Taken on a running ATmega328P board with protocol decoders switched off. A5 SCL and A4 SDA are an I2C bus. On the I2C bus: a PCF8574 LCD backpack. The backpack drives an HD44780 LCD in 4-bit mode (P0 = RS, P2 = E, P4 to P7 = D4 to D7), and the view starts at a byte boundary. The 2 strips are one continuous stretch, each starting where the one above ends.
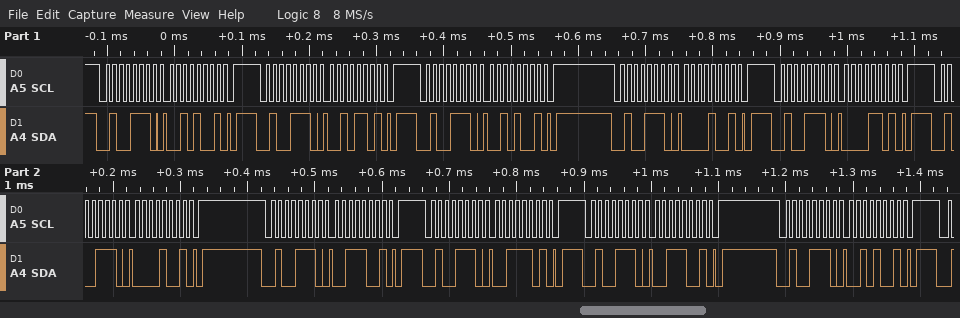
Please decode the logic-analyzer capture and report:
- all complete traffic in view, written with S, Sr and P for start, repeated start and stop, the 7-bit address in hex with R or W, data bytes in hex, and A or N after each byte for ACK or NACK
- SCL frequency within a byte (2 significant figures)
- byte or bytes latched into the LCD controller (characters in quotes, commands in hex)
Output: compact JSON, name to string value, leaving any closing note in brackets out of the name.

{"all complete traffic in view, written with S, Sr and P for start, repeated start and stop, the 7-bit address in hex with R or W, data bytes in hex, and A or N after each byte for ACK or NACK": "S 27W A 29 A P S 27W A 2D A P S 27W A 29 A P S 27W A 09 A P S 27W A 0D A P S 27W A 09 A P S 27W A 39 A P S 27W A 3D A P S 27W A 39 A P S 27W A 29 A P", "SCL frequency within a byte": "100 kHz", "byte or bytes latched into the LCD controller": "' '"}
